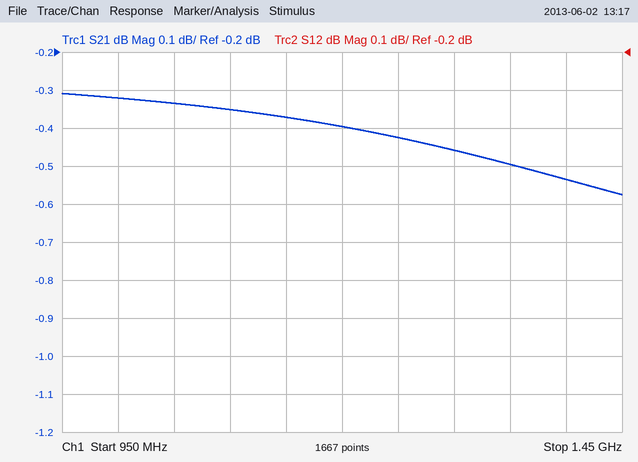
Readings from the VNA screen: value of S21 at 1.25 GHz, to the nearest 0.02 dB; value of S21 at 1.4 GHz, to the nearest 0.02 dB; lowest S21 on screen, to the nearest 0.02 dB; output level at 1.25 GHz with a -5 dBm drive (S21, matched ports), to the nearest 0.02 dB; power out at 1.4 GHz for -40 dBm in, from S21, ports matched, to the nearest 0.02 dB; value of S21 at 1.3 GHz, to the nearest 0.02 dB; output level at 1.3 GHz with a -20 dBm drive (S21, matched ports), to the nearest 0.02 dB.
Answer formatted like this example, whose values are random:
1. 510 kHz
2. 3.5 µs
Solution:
1. -0.42 dB
2. -0.54 dB
3. -0.58 dB
4. -5.42 dBm
5. -40.54 dBm
6. -0.46 dB
7. -20.46 dBm
